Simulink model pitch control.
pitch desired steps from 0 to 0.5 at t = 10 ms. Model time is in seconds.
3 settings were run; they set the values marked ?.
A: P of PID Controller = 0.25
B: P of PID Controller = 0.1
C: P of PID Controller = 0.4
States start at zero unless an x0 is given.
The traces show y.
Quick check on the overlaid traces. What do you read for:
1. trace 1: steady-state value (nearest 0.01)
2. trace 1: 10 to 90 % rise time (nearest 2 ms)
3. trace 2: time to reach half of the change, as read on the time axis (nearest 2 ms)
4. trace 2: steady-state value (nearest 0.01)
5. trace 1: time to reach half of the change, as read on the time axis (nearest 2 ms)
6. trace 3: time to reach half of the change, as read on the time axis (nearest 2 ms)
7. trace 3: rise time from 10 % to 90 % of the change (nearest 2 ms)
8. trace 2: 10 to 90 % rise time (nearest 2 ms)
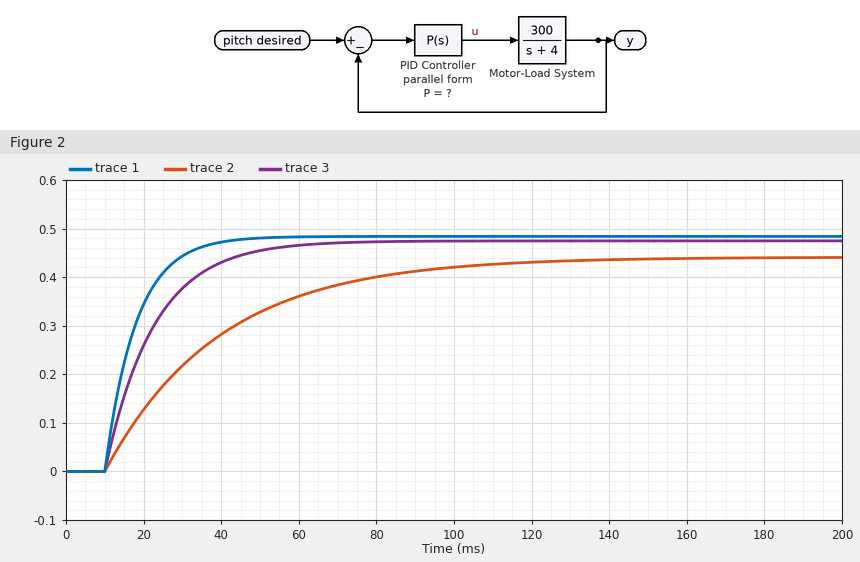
0.48
18 ms
30 ms
0.44
16 ms
18 ms
28 ms
64 ms
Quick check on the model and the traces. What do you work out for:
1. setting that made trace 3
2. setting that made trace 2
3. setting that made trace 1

A
B
C
